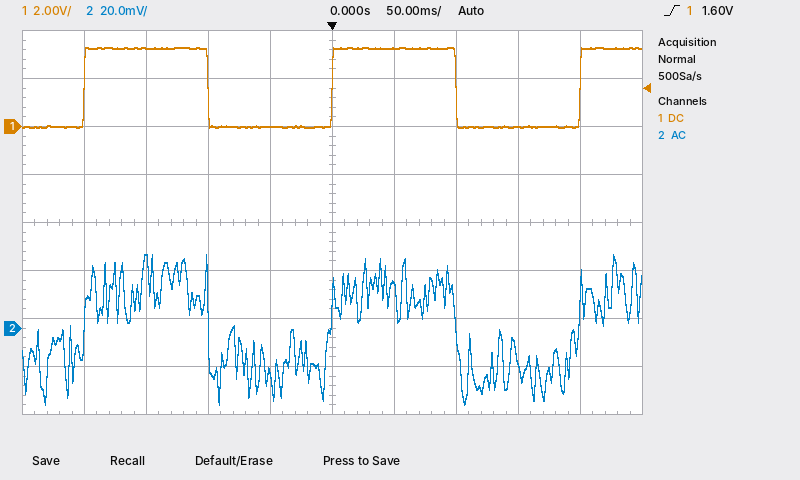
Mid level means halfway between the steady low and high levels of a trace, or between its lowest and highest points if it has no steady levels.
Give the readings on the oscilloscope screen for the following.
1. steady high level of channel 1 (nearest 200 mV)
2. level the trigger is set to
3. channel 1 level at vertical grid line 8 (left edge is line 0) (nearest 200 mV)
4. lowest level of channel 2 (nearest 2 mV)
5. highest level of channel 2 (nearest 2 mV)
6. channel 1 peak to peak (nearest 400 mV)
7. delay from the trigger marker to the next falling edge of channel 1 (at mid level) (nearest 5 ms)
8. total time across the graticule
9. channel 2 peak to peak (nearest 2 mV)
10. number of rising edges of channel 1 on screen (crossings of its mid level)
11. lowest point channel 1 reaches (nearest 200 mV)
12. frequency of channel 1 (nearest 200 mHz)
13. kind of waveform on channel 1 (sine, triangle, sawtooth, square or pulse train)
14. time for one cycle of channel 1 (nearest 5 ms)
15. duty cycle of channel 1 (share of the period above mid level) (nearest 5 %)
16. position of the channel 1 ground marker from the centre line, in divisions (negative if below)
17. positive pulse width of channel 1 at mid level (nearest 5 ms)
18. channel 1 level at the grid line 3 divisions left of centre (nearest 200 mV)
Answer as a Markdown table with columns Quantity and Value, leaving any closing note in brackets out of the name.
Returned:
| Quantity | Value |
|---|---|
| steady high level of channel 1 | 3.2 V |
| level the trigger is set to | 1.60 V |
| channel 1 level at vertical grid line 8 (left edge is line 0) | 0.0 V |
| lowest level of channel 2 | -32 mV |
| highest level of channel 2 | 30 mV |
| channel 1 peak to peak | 3.2 V |
| delay from the trigger marker to the next falling edge of channel 1 (at mid level) | 100 ms |
| total time across the graticule | 500 ms |
| channel 2 peak to peak | 62 mV |
| number of rising edges of channel 1 on screen | 3 |
| lowest point channel 1 reaches | 0.0 V |
| frequency of channel 1 | 5.0 Hz |
| kind of waveform on channel 1 | square |
| time for one cycle of channel 1 | 200 ms |
| duty cycle of channel 1 (share of the period above mid level) | 50 % |
| position of the channel 1 ground marker from the centre line, in divisions | +2.0 div |
| positive pulse width of channel 1 at mid level | 100 ms |
| channel 1 level at the grid line 3 divisions left of centre | 3.2 V |
